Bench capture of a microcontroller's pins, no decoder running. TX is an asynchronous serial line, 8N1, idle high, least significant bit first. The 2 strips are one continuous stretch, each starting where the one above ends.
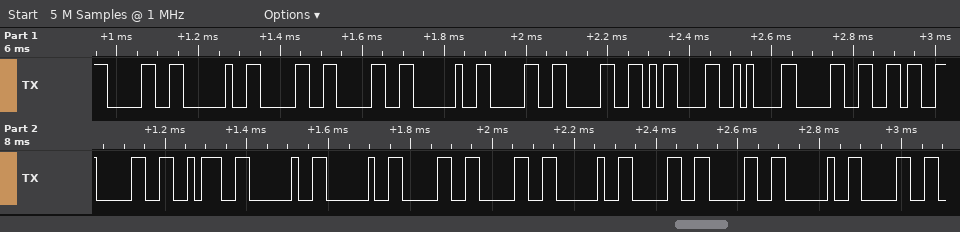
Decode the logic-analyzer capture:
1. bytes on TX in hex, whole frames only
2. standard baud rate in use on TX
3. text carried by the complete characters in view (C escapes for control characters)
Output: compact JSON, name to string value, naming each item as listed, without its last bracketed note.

{"bytes on TX in hex, whole frames only": "30 20 30 30 20 30 30 0D 0A 30 36 30 3A 20 20 30 30 20 30 30 20 30", "standard baud rate in use on TX": "57600 baud", "text carried by the complete characters in view": "\"0 00 00\\r\\n060:  00 00 0\""}
